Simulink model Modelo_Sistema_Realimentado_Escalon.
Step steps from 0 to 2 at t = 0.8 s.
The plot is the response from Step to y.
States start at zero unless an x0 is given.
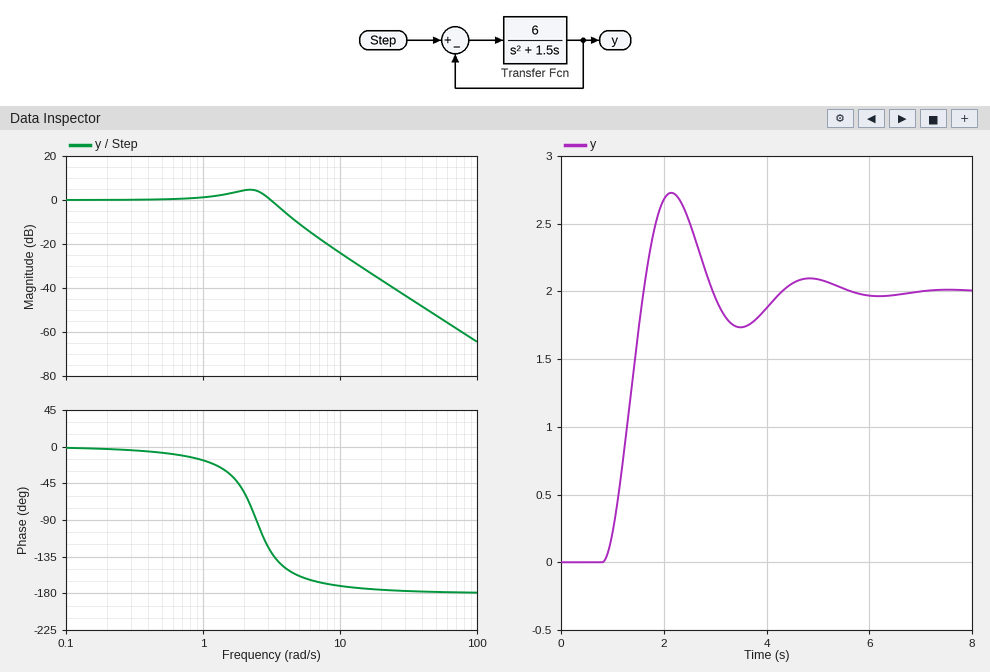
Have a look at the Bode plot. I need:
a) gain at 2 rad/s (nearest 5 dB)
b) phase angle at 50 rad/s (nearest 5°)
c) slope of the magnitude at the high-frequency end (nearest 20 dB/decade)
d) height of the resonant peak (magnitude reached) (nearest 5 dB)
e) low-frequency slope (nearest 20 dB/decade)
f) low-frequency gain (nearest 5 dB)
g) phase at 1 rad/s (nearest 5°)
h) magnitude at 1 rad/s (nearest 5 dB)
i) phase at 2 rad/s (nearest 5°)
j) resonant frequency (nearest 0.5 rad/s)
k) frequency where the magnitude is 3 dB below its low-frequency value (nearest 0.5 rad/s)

5 dB
-180°
-40 dB/decade
5 dB
0 dB/decade
0 dB
-15°
0 dB
-55°
2.0 rad/s
3.5 rad/s
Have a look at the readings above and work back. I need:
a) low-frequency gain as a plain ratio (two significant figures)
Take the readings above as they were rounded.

1.0
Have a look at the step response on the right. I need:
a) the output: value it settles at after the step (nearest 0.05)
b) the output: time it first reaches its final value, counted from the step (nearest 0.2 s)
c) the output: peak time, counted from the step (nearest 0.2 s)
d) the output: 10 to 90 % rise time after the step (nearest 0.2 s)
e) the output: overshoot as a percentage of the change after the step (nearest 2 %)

2.00
0.8 s
1.4 s
0.6 s
36 %
